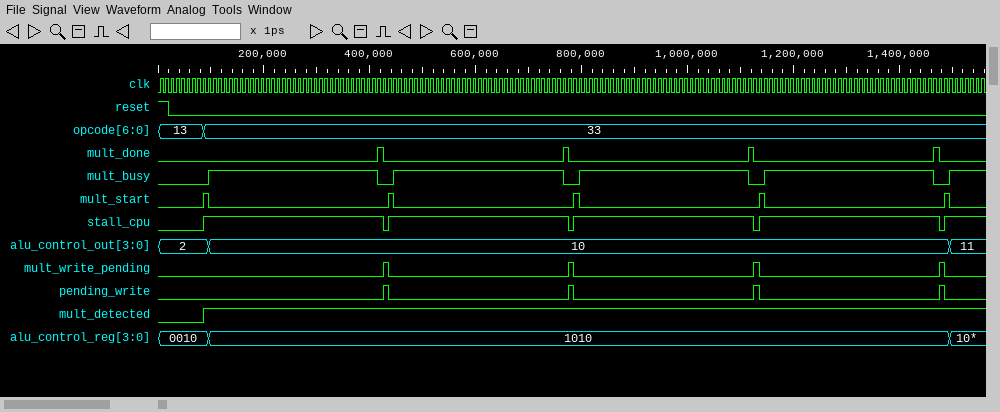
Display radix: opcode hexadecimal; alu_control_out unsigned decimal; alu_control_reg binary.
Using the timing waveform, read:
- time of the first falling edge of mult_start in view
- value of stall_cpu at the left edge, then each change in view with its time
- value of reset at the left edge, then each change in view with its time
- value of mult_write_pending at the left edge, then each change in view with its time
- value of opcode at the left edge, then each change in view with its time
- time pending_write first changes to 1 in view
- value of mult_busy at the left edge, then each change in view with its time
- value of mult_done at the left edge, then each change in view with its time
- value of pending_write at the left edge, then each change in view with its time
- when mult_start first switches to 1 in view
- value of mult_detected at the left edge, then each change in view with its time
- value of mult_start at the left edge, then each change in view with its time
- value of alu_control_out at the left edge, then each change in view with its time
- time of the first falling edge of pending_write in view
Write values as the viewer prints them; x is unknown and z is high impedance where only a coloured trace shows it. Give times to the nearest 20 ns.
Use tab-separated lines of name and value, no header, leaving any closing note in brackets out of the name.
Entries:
time of the first falling edge of mult_start in view	100 ns
value of stall_cpu at the left edge, then each change in view with its time	0, 1 at 80 ns, 0 at 420 ns, 1 at 440 ns, 0 at 780 ns, 1 at 780 ns, 0 at 1120 ns, 1 at 1140 ns, 0 at 1480 ns, 1 at 1480 ns
value of reset at the left edge, then each change in view with its time	1, 0 at 20 ns
value of mult_write_pending at the left edge, then each change in view with its time	0, 1 at 420 ns, 0 at 440 ns, 1 at 780 ns, 0 at 780 ns, 1 at 1120 ns, 0 at 1140 ns, 1 at 1480 ns, 0 at 1480 ns
value of opcode at the left edge, then each change in view with its time	13, 33 at 80 ns
time pending_write first changes to 1 in view	420 ns
value of mult_busy at the left edge, then each change in view with its time	0, 1 at 100 ns, 0 at 420 ns, 1 at 440 ns, 0 at 760 ns, 1 at 800 ns, 0 at 1120 ns, 1 at 1140 ns, 0 at 1460 ns, 1 at 1500 ns
value of mult_done at the left edge, then each change in view with its time	0, 1 at 420 ns, 0 at 420 ns, 1 at 760 ns, 0 at 780 ns, 1 at 1120 ns, 0 at 1120 ns, 1 at 1460 ns, 0 at 1480 ns
value of pending_write at the left edge, then each change in view with its time	0, 1 at 420 ns, 0 at 440 ns, 1 at 780 ns, 0 at 780 ns, 1 at 1120 ns, 0 at 1140 ns, 1 at 1480 ns, 0 at 1480 ns
when mult_start first switches to 1 in view	80 ns
value of mult_detected at the left edge, then each change in view with its time	0, 1 at 80 ns
value of mult_start at the left edge, then each change in view with its time	0, 1 at 80 ns, 0 at 100 ns, 1 at 440 ns, 0 at 440 ns, 1 at 780 ns, 0 at 800 ns, 1 at 1140 ns, 0 at 1140 ns, 1 at 1480 ns, 0 at 1500 ns
value of alu_control_out at the left edge, then each change in view with its time	2, 10 at 100 ns, 11 at 1500 ns
time of the first falling edge of pending_write in view	440 ns
